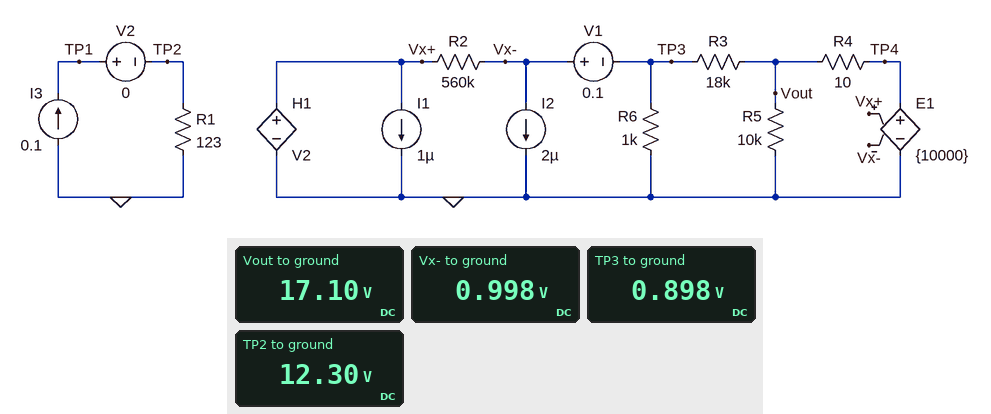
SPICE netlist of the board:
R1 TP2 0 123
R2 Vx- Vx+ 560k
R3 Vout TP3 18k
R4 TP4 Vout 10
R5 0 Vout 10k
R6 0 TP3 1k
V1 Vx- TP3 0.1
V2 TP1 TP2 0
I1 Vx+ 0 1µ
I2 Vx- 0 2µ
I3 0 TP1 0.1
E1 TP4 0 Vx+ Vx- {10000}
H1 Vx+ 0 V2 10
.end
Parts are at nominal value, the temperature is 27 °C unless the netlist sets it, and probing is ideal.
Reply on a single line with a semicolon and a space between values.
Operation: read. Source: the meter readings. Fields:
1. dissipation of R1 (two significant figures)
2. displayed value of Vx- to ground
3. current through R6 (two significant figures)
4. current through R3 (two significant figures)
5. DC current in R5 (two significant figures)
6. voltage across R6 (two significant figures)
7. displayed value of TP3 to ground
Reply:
1.2 W; 0.998 V; 900 µA; 900 µA; 1.7 mA; 900 mV; 0.898 V
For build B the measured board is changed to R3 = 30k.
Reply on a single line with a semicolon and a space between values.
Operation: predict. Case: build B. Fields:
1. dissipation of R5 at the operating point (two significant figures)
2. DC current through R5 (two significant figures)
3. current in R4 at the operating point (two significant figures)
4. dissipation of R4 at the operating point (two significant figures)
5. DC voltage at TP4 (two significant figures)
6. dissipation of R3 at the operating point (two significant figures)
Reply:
78 mW; 2.8 mA; 3.7 mA; 140 µW; 28 V; 24 mW
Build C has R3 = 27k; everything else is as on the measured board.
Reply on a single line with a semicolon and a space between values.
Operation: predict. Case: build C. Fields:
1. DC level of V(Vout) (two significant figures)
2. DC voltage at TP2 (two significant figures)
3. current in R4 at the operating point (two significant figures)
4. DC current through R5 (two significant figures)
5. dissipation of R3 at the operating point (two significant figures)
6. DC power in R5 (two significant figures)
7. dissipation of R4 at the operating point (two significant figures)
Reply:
25 V; 12 V; 3.4 mA; 2.5 mA; 22 mW; 63 mW; 120 µW
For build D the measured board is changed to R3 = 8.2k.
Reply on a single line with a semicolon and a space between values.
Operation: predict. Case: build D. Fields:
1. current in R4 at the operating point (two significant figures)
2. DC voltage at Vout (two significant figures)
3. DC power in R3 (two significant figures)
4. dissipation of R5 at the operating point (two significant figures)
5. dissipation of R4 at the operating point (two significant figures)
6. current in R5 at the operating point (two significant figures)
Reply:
1.7 mA; 8.3 V; 6.7 mW; 6.9 mW; 30 µW; 830 µA
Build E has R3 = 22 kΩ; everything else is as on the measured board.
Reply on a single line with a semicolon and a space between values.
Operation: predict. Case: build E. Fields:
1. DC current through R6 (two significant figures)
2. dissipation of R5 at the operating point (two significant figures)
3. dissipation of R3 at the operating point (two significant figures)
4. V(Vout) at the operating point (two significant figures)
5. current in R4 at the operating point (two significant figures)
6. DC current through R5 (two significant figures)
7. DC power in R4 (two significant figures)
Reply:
900 µA; 43 mW; 18 mW; 21 V; 3.0 mA; 2.1 mA; 88 µW
